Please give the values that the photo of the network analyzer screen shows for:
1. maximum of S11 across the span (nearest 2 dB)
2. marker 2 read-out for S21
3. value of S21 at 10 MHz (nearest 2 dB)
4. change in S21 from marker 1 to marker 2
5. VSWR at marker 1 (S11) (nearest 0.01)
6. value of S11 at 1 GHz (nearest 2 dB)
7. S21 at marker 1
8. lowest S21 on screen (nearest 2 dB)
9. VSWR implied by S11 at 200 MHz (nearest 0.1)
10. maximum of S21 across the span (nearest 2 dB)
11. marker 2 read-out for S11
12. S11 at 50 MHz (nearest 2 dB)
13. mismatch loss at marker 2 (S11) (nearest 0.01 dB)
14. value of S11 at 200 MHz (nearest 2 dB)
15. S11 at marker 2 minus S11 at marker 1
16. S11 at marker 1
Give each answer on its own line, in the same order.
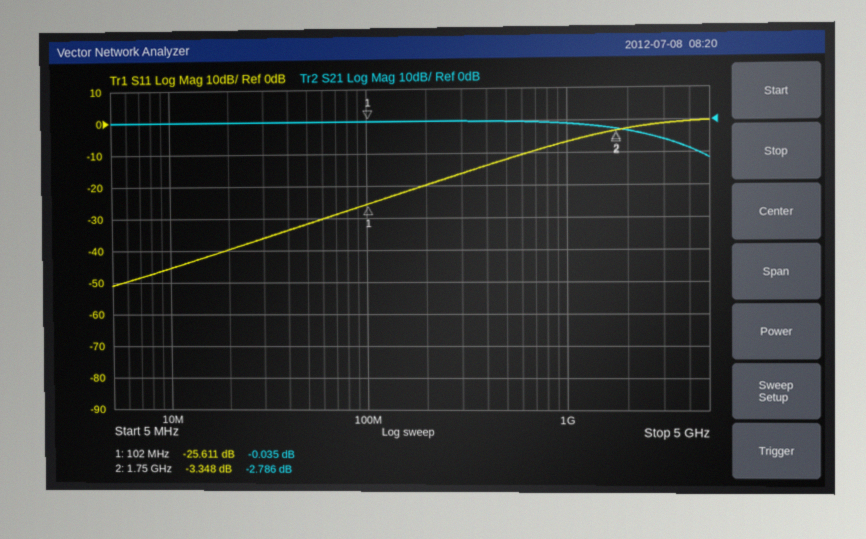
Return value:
0 dB
-2.786 dB
0 dB
-2.751 dB
1.11
-6 dB
-0.035 dB
-12 dB
1.2
0 dB
-3.348 dB
-32 dB
2.70 dB
-20 dB
22.263 dB
-25.611 dB
